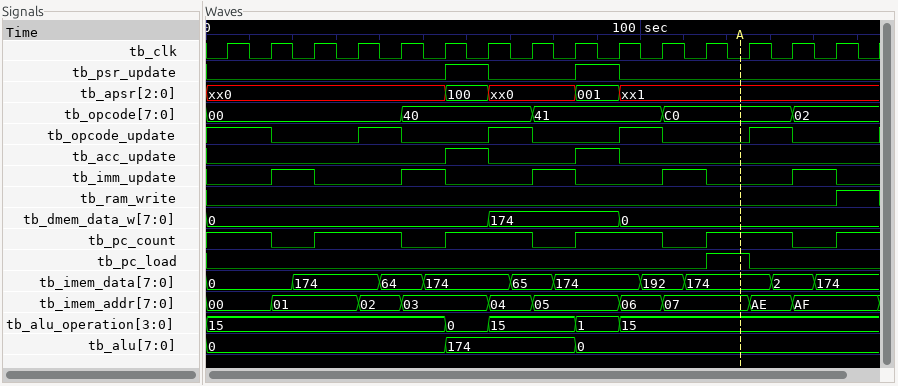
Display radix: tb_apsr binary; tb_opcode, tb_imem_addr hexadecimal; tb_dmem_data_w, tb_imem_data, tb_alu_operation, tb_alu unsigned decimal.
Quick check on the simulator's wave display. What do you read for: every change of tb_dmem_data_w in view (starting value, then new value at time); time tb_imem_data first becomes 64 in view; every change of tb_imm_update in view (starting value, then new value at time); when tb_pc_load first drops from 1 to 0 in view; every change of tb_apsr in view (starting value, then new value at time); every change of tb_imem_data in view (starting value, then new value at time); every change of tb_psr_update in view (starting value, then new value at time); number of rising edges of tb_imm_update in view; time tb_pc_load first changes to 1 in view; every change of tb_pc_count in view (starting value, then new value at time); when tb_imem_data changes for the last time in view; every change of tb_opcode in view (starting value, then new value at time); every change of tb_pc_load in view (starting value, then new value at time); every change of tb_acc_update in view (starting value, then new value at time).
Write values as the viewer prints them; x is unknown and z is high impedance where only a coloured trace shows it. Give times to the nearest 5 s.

0, 174 at 65 s, 0 at 95 s
40 s
0, 1 at 15 s, 0 at 25 s, 1 at 45 s, 0 at 55 s, 1 at 75 s, 0 at 85 s, 1 at 105 s, 0 at 115 s, 1 at 135 s, 0 at 145 s
125 s
xx0, 100 at 55 s, xx0 at 65 s, 001 at 85 s, xx1 at 95 s
0, 174 at 20 s, 64 at 40 s, 174 at 50 s, 65 at 70 s, 174 at 80 s, 192 at 100 s, 174 at 110 s, 2 at 130 s, 174 at 140 s
0, 1 at 55 s, 0 at 65 s, 1 at 85 s, 0 at 95 s
5
115 s
1, 0 at 15 s, 1 at 25 s, 0 at 45 s, 1 at 55 s, 0 at 75 s, 1 at 85 s, 0 at 105 s, 1 at 115 s, 0 at 135 s, 1 at 145 s
140 s
00, 40 at 45 s, 41 at 75 s, C0 at 105 s, 02 at 135 s
0, 1 at 115 s, 0 at 125 s
0, 1 at 55 s, 0 at 65 s, 1 at 85 s, 0 at 95 s
